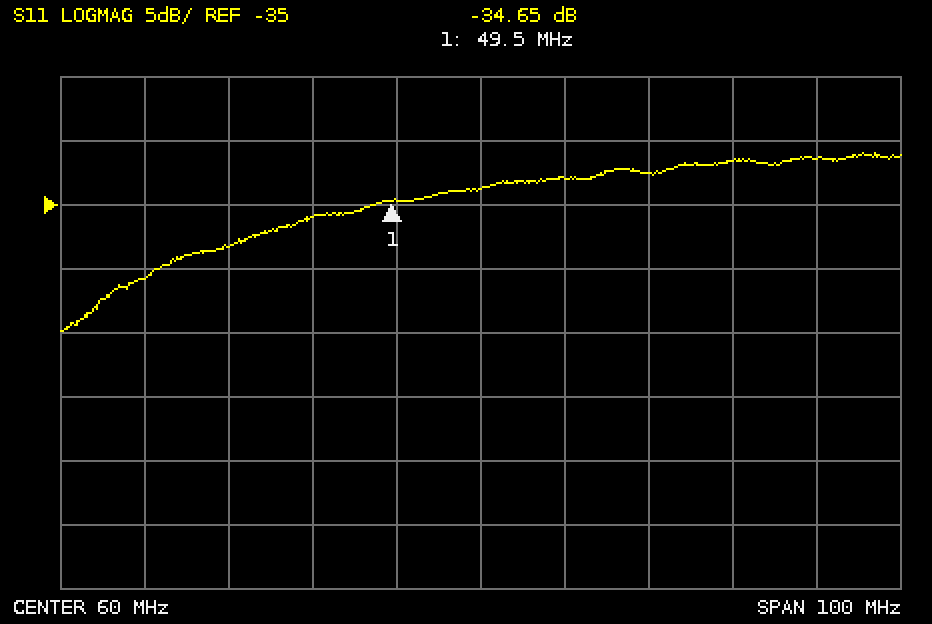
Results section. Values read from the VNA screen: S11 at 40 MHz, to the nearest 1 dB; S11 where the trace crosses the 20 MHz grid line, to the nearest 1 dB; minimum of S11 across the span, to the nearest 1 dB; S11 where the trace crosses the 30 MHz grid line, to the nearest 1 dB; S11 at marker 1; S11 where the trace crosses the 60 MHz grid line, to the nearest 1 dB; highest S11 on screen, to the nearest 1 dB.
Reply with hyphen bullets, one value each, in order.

- -36 dB
- -41 dB
- -45 dB
- -38 dB
- -34.65 dB
- -34 dB
- -31 dB
